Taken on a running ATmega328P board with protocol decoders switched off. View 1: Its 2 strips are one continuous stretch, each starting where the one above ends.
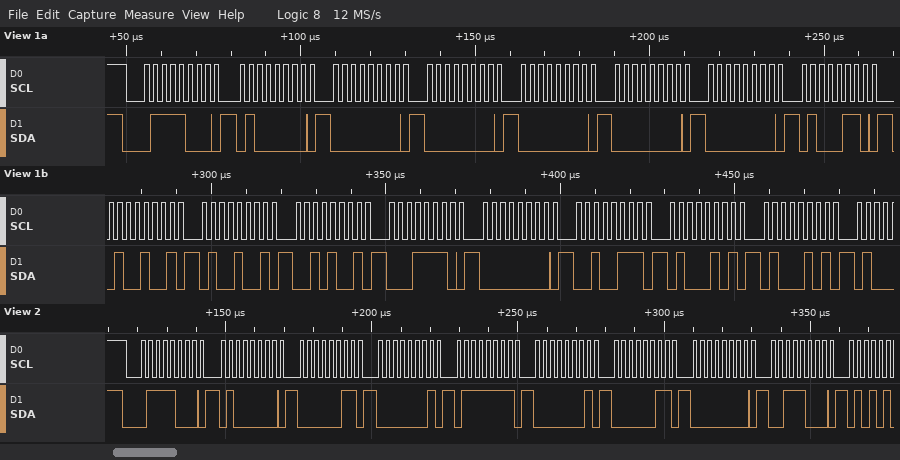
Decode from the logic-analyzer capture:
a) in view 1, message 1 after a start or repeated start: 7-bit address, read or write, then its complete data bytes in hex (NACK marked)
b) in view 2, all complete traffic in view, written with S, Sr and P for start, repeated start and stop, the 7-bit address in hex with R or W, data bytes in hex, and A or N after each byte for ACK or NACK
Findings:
0x3C write: 40 00 00 00 00 00 46 49 49 29 1E 00 27 45 45
S 3CW A 40 A 03 A 01 A 7F A 01 A 03 A 00 A 38 A
